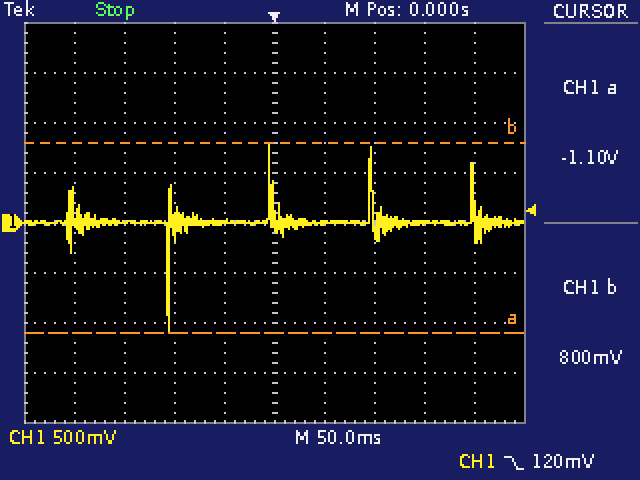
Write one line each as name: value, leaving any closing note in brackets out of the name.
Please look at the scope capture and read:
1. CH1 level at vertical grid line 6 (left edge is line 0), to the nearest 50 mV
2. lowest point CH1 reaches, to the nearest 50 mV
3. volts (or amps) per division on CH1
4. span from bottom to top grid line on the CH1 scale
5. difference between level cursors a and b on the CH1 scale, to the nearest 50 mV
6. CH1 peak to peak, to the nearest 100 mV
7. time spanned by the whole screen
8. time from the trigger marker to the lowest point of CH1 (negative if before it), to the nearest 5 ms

CH1 level at vertical grid line 6 (left edge is line 0), to the nearest 50 mV: 0 mV
lowest point CH1 reaches, to the nearest 50 mV: -1.10 V
volts (or amps) per division on CH1: 500 mV
span from bottom to top grid line on the CH1 scale: 4 V
difference between level cursors a and b on the CH1 scale, to the nearest 50 mV: 1.90 V
CH1 peak to peak, to the nearest 100 mV: 1.90 V
time spanned by the whole screen: 500 ms
time from the trigger marker to the lowest point of CH1 (negative if before it), to the nearest 5 ms: -105 ms
